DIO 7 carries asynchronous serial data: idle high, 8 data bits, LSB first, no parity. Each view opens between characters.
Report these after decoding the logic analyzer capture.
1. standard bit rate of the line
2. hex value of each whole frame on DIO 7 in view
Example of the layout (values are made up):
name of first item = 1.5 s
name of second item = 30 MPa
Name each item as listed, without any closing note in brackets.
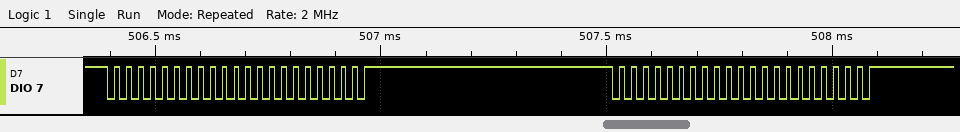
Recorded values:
standard bit rate of the line = 74880 baud
hex value of each whole frame on DIO 7 in view = 55, 55, 55, 55, FD, 55, 55, 55, 55, FD
